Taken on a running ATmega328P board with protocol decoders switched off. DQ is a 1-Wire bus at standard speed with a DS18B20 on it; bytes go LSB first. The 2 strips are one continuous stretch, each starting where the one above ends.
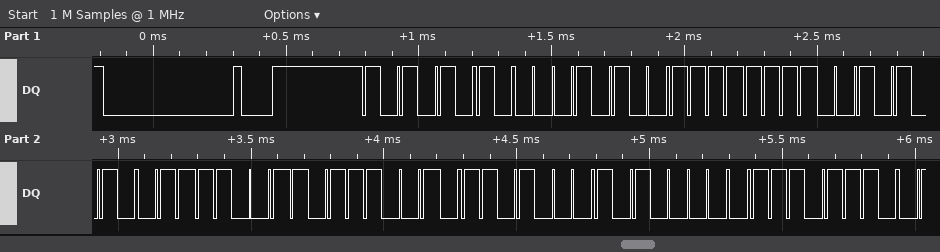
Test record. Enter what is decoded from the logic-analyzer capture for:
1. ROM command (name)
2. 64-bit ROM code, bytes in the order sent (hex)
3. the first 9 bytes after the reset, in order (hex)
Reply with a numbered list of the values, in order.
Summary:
1. Match ROM
2. 28 FF 54 9E 9D 16 05 77
3. 55 28 FF 54 9E 9D 16 05 77
